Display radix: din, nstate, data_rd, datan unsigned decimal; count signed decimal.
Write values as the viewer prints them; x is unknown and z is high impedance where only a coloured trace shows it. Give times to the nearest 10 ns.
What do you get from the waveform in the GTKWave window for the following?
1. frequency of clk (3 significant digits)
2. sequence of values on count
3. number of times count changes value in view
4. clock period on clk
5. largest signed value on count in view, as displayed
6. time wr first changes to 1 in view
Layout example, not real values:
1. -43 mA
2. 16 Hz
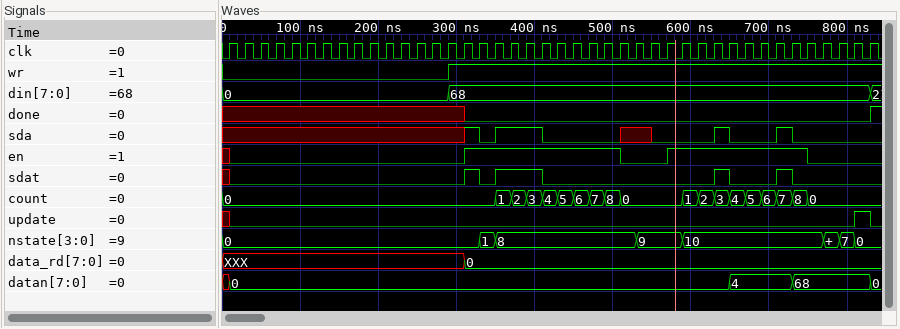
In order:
1. 50.0 MHz
2. 0, 1, 2, 3, 4, 5, 6, 7, 8, 0, 1, 2, 3, 4, 5, 6, 7, 8, 0
3. 18
4. 20 ns
5. 8
6. 290 ns
